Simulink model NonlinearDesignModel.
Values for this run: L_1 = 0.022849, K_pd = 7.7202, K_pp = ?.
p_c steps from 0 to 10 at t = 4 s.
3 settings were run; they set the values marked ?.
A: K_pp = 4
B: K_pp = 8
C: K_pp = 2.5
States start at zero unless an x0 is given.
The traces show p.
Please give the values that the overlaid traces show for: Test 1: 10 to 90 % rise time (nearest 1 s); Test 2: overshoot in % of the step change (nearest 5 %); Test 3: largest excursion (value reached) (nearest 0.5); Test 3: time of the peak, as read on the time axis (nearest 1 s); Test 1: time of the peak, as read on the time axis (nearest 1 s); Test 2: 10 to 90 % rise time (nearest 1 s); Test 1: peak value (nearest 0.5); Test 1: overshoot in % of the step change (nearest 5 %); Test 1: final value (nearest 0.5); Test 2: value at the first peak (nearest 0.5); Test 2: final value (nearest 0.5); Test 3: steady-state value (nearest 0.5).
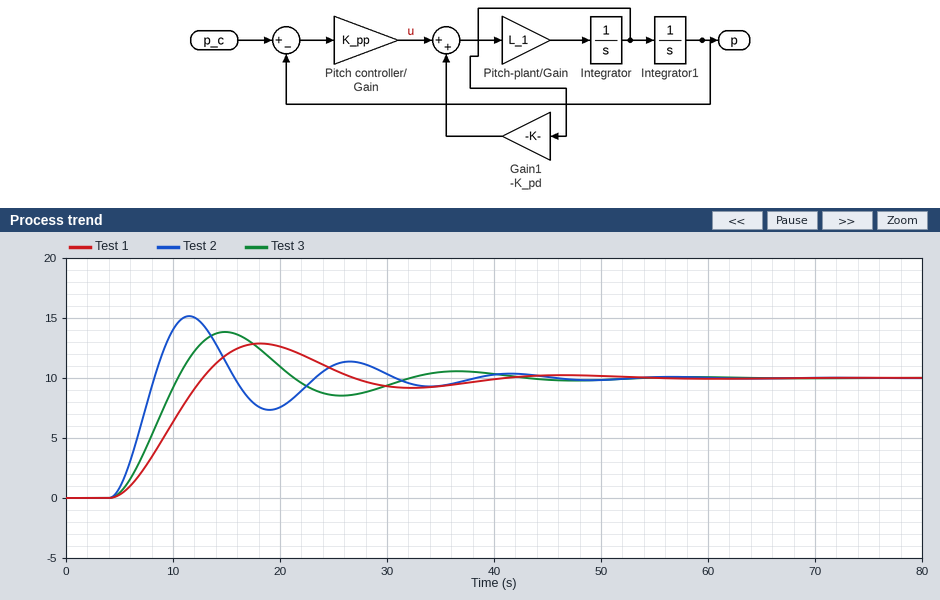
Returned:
6 s
50 %
14.0
15 s
18 s
3 s
13.0
30 %
10.0
15.0
10.0
10.0
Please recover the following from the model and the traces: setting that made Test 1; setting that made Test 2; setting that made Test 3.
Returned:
C
B
A
